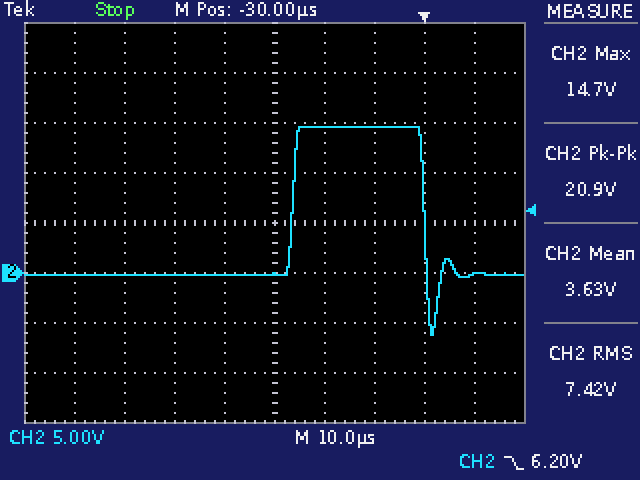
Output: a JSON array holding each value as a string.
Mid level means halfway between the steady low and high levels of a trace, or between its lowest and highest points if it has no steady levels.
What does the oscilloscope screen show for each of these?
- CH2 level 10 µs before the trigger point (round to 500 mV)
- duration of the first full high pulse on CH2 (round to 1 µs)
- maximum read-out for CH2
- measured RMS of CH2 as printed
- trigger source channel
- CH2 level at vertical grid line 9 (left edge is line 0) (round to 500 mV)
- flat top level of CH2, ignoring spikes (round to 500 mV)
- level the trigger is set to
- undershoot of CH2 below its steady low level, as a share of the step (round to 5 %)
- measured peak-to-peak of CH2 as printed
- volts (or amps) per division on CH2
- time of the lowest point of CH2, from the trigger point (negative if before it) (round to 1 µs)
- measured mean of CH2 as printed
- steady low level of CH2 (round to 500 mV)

["14.5 V", "26 µs", "14.7 V", "7.42 V", "CH2", "0.0 V", "14.5 V", "6.20 V", "40 %", "20.9 V", "5 V", "+2 µs", "3.63 V", "0.0 V"]
